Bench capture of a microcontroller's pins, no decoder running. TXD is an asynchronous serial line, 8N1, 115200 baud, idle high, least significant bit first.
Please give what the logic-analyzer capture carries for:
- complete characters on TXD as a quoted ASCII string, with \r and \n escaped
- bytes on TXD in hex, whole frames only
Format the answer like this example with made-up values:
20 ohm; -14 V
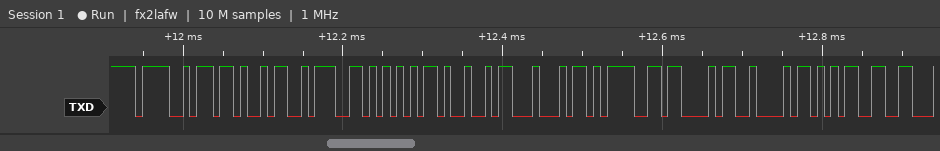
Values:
"OK:UID=CB5"; 0x4F 0x4B 0x3A 0x55 0x49 0x44 0x3D 0x43 0x42 0x35
